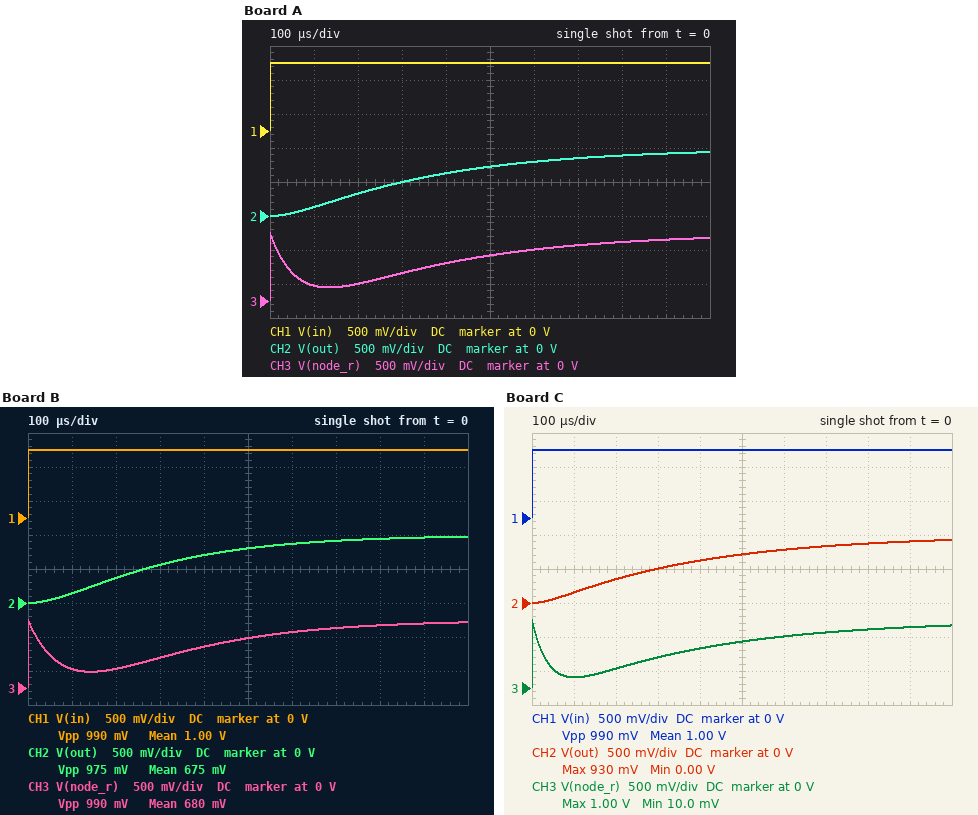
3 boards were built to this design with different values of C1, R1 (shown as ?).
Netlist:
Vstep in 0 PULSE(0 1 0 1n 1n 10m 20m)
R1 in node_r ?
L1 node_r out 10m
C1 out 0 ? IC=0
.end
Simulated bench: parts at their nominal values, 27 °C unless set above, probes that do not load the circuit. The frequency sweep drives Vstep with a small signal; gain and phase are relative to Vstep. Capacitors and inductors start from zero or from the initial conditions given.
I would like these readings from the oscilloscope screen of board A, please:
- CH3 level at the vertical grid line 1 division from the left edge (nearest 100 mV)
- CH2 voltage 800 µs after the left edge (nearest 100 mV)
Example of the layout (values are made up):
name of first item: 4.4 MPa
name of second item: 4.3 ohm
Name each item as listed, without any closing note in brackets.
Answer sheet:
CH3 level at the vertical grid line 1 division from the left edge: 200 mV
CH2 voltage 800 µs after the left edge: 900 mV
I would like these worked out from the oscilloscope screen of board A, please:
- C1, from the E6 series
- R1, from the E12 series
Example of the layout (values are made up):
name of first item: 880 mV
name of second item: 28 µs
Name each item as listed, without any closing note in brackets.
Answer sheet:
C1, from the E6 series: 2.2 µF
R1, from the E12 series: 180 Ω
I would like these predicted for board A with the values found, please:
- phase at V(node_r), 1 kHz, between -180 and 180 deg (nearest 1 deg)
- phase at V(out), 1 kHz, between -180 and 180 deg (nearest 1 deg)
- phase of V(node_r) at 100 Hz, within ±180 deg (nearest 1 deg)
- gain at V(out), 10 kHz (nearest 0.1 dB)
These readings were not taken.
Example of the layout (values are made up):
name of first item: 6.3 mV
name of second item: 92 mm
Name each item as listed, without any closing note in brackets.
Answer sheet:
phase at V(node_r), 1 kHz, between -180 and 180 deg: -87 deg
phase at V(out), 1 kHz, between -180 and 180 deg: -87 deg
phase of V(node_r) at 100 Hz, within ±180 deg: -14 deg
gain at V(out), 10 kHz: -39.0 dB
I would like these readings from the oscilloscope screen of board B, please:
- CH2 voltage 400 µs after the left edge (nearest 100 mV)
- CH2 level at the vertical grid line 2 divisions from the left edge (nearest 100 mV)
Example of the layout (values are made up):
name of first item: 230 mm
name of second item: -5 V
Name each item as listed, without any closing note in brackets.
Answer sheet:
CH2 voltage 400 µs after the left edge: 700 mV
CH2 level at the vertical grid line 2 divisions from the left edge: 400 mV
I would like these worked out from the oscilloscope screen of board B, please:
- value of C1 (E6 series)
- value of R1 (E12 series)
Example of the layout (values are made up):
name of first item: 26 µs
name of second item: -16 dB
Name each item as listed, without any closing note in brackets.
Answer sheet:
value of C1: 2.2 µF
value of R1: 150 Ω
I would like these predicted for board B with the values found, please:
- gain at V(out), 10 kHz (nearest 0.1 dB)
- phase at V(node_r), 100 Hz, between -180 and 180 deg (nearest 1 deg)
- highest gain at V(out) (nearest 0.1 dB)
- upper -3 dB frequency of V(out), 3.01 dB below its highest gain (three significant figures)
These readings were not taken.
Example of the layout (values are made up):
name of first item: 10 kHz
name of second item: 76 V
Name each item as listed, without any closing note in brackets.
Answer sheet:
gain at V(out), 10 kHz: -38.9 dB
phase at V(node_r), 100 Hz, between -180 and 180 deg: -12 deg
highest gain at V(out): 0 dB
upper -3 dB frequency of V(out), 3.01 dB below its highest gain: 595 Hz
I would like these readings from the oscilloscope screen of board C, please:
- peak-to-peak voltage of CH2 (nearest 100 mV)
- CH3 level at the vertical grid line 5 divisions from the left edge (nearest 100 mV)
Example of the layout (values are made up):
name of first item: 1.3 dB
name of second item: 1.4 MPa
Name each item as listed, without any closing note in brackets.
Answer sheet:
peak-to-peak voltage of CH2: 900 mV
CH3 level at the vertical grid line 5 divisions from the left edge: 700 mV
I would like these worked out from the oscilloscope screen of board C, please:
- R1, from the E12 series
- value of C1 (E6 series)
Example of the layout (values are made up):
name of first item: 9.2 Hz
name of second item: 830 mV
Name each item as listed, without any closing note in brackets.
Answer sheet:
R1, from the E12 series: 270 Ω
value of C1: 1.5 µF
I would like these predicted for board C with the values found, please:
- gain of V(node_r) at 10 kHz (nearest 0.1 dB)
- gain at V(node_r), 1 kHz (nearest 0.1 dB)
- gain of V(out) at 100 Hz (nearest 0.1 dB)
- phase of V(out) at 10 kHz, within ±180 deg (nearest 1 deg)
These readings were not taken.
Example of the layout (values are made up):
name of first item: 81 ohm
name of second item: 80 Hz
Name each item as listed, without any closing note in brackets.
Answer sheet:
gain of V(node_r) at 10 kHz: -0.8 dB
gain at V(node_r), 1 kHz: -16.0 dB
gain of V(out) at 100 Hz: -0.2 dB
phase of V(out) at 10 kHz, within ±180 deg: -156 deg
